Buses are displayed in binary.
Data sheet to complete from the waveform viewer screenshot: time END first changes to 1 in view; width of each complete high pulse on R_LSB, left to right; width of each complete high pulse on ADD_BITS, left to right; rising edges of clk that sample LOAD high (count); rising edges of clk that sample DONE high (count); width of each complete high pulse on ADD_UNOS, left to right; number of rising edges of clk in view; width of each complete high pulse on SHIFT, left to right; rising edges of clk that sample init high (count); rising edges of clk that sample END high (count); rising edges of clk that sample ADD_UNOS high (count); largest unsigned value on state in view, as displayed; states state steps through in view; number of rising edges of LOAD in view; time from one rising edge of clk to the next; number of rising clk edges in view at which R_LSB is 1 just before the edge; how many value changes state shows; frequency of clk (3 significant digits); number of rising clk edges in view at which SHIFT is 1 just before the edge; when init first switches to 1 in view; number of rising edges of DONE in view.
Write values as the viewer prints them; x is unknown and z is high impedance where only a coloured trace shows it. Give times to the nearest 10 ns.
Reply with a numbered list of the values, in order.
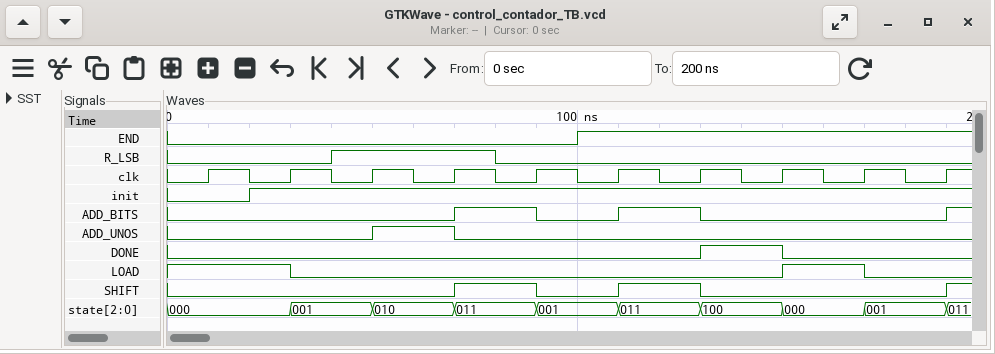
1. 100 ns
2. 40 ns
3. 20 ns, 20 ns
4. 3
5. 1
6. 20 ns
7. 10
8. 20 ns, 20 ns
9. 9
10. 5
11. 1
12. 100
13. 000, 001, 010, 011, 001, 011, 100, 000, 001, 011
14. 1
15. 20 ns
16. 2
17. 9
18. 50.0 MHz
19. 2
20. 20 ns
21. 1
